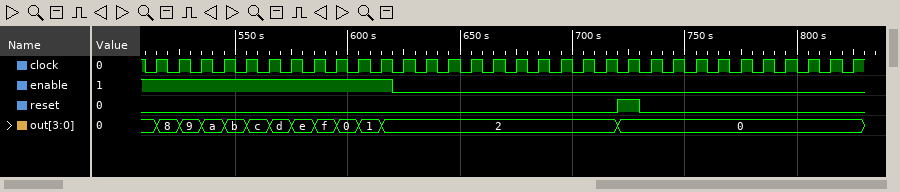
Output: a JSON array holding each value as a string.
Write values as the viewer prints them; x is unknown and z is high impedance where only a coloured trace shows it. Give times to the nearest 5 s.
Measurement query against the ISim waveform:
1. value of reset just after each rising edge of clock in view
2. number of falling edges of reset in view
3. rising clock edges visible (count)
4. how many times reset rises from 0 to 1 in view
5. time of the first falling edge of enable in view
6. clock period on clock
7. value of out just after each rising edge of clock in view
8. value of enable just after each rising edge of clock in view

["0 0 0 0 0 0 0 0 0 0 0 0 0 0 0 0 0 0 0 0 0 1 0 0 0 0 0 0 0 0 0 0", "1", "32", "1", "620 s", "10 s", "8, 9, a, b, c, d, e, f, 0, 1, 2, 2, 2, 2, 2, 2, 2, 2, 2, 2, 2, 0, 0, 0, 0, 0, 0, 0, 0, 0, 0, 0", "1 1 1 1 1 1 1 1 1 1 1 0 0 0 0 0 0 0 0 0 0 0 0 0 0 0 0 0 0 0 0 0"]
